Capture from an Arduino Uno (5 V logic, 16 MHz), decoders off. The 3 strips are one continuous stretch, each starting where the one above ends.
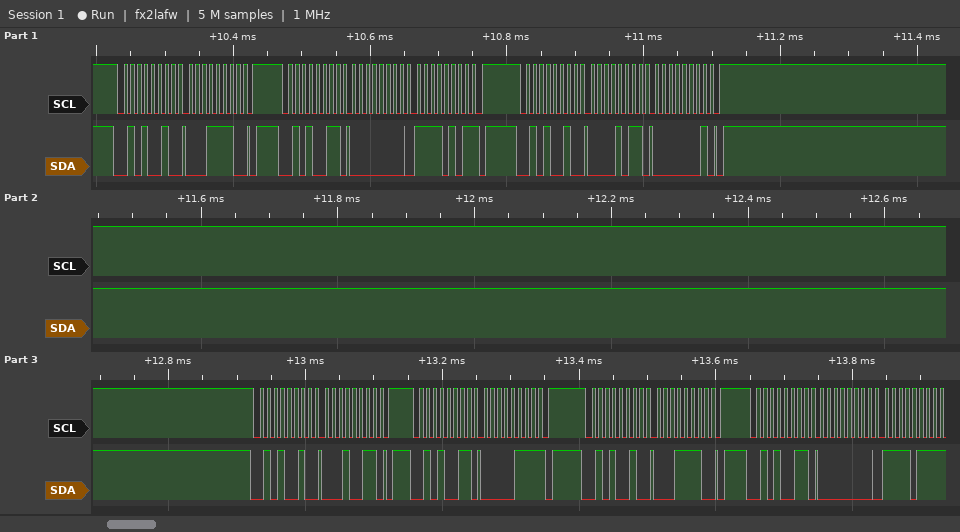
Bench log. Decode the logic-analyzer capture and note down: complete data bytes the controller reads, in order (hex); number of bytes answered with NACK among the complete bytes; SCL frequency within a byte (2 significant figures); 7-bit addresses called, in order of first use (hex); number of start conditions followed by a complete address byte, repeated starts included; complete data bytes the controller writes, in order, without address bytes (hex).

00 F5 07 00 F7
3
100 kHz
0x29
7
1E 0B 01 13 1E
